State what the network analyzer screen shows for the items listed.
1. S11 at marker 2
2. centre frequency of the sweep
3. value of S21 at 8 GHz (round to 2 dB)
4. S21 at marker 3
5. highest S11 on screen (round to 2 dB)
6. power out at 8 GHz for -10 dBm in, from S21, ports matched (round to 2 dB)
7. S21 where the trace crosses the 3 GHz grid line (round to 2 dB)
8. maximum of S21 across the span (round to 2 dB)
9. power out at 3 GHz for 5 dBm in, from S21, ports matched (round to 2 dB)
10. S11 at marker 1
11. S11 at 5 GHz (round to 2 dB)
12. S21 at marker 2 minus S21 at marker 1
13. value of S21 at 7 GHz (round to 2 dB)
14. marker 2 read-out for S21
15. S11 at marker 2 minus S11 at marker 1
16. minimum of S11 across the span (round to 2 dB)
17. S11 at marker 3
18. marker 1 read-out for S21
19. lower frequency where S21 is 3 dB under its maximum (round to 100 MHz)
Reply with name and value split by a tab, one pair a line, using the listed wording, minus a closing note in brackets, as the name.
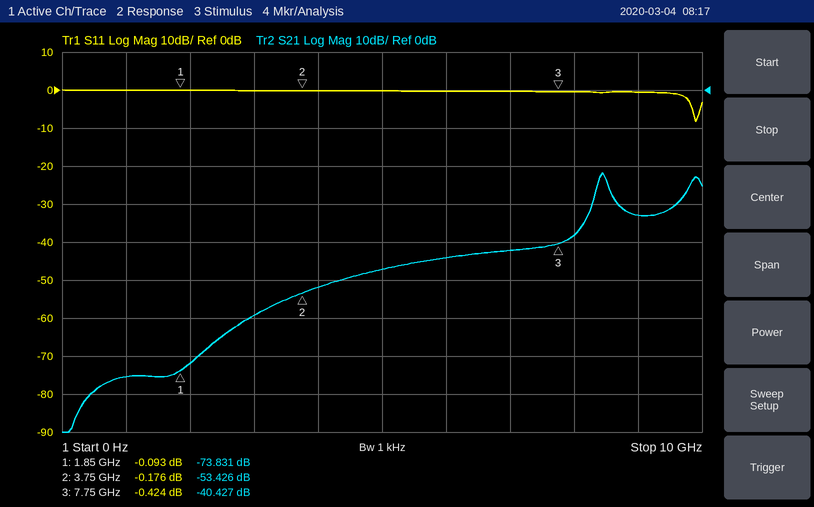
S11 at marker 2	-0.176 dB
centre frequency of the sweep	5 GHz
value of S21 at 8 GHz	-38 dB
S21 at marker 3	-40.427 dB
highest S11 on screen	0 dB
power out at 8 GHz for -10 dBm in, from S21, ports matched	-48 dBm
S21 where the trace crosses the 3 GHz grid line	-60 dB
maximum of S21 across the span	-22 dB
power out at 3 GHz for 5 dBm in, from S21, ports matched	-54 dBm
S11 at marker 1	-0.093 dB
S11 at 5 GHz	0 dB
S21 at marker 2 minus S21 at marker 1	20.405 dB
value of S21 at 7 GHz	-42 dB
marker 2 read-out for S21	-53.426 dB
S11 at marker 2 minus S11 at marker 1	-0.083 dB
minimum of S11 across the span	-8 dB
S11 at marker 3	-0.424 dB
marker 1 read-out for S21	-73.831 dB
lower frequency where S21 is 3 dB under its maximum	8.4 GHz
